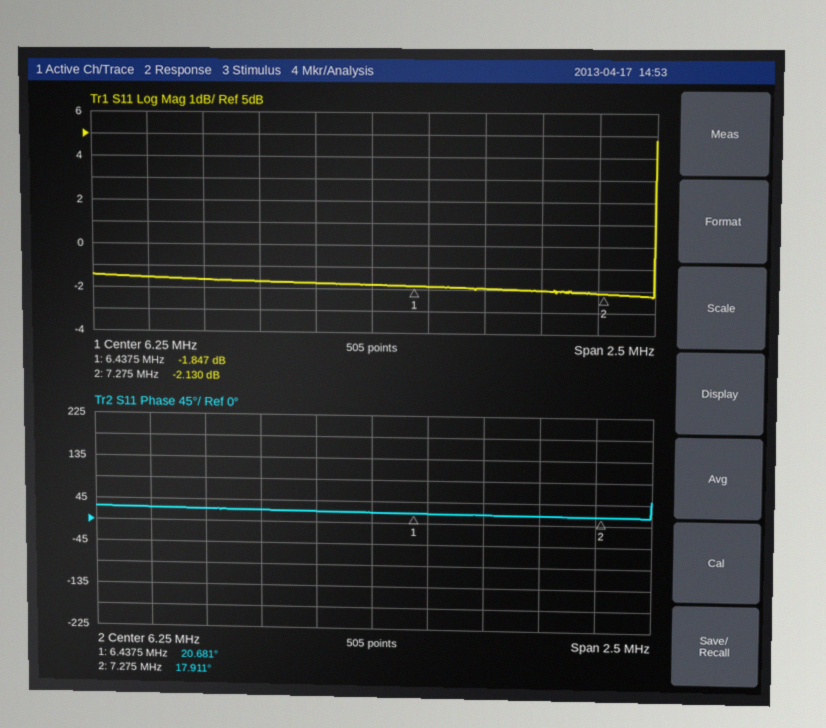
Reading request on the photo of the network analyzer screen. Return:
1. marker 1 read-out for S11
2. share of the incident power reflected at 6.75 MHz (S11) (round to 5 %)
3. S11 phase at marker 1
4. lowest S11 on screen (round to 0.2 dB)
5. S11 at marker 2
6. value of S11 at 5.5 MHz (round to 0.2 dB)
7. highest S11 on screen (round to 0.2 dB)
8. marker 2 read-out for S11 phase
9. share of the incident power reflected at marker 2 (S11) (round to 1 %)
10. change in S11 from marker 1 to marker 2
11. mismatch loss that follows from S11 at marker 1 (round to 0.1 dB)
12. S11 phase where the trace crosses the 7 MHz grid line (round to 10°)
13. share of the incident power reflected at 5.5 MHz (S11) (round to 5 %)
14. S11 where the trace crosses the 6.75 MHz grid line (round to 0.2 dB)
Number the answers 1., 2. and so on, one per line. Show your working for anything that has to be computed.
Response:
1. -1.847 dB
2. 10^(-2/10) ≈ 63.1 %, so 65 % to the nearest 5 %
3. 20.681°
4. -2.2 dB
5. -2.130 dB
6. -1.6 dB
7. 4.8 dB
8. 17.911°
9. 10^(-2.13/10) ≈ 61 %
10. -2.13 − (-1.847) = -0.283 dB
11. −10 log10(1 − 10^(-1.847/10)) ≈ 4.6 dB
12. 20°
13. 10^(-1.6/10) ≈ 69.2 %, so 70 % to the nearest 5 %
14. -2.0 dB
